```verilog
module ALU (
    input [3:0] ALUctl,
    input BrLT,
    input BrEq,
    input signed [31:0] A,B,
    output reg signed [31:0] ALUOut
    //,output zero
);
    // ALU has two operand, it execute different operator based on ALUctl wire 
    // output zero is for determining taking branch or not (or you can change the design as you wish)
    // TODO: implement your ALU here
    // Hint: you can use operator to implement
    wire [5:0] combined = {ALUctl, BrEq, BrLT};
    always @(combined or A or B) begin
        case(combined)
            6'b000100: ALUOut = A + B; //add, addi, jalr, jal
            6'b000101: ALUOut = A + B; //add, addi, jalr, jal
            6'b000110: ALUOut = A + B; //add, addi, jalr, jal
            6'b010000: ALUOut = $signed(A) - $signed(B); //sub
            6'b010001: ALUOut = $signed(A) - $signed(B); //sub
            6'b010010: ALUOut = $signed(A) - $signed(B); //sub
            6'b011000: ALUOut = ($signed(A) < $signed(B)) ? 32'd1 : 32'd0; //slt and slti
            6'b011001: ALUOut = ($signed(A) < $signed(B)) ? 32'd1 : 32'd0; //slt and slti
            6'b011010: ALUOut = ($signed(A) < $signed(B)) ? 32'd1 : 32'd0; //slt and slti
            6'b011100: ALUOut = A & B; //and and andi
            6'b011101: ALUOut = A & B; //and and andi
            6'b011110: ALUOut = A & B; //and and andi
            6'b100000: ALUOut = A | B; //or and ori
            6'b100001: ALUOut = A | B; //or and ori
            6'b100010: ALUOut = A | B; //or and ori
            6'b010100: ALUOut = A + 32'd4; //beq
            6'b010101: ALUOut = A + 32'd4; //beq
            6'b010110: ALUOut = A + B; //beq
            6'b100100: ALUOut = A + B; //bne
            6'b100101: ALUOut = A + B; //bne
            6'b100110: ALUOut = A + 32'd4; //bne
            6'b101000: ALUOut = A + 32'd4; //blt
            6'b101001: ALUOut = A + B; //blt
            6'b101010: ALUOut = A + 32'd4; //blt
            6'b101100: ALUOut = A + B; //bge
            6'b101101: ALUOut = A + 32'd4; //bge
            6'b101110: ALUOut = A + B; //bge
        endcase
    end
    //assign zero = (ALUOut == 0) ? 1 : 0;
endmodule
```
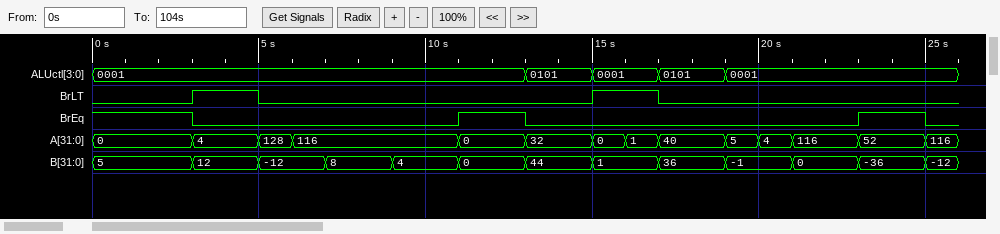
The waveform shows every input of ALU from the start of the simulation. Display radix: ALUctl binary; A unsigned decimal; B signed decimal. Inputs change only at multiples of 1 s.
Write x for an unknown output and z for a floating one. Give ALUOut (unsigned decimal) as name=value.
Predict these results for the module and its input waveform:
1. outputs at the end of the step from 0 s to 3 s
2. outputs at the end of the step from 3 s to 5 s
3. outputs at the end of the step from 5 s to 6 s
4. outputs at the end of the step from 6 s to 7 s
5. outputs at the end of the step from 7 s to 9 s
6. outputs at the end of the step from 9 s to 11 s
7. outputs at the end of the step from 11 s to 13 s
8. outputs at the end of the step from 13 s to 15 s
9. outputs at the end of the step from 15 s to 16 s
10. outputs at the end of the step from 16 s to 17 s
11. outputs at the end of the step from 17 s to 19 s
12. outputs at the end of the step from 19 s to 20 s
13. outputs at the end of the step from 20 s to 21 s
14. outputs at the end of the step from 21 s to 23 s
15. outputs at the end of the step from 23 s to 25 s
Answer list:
ALUOut=5
ALUOut=16
ALUOut=116
ALUOut=104
ALUOut=124
ALUOut=120
ALUOut=0
ALUOut=36
ALUOut=1
ALUOut=2
ALUOut=44
ALUOut=4
ALUOut=3
ALUOut=116
ALUOut=16
